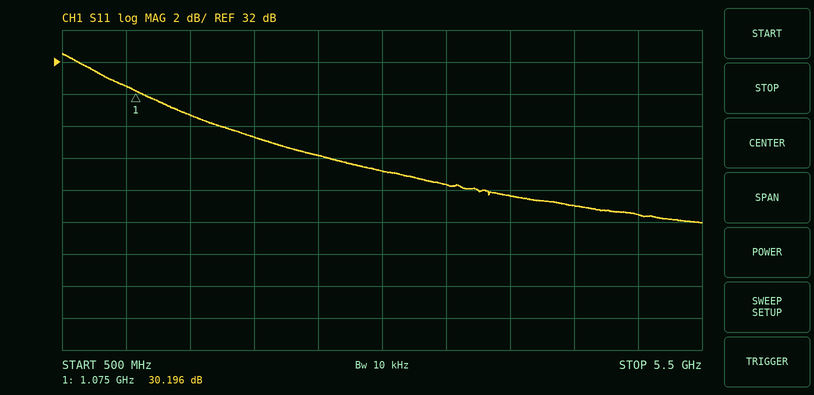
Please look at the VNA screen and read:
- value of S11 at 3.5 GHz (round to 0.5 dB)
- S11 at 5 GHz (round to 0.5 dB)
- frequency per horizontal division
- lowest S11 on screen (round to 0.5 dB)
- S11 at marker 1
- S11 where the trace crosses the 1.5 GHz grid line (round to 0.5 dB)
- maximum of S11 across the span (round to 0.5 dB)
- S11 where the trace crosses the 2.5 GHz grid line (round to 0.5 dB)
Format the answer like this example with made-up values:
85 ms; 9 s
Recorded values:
24.5 dB; 22.5 dB; 500 MHz; 22.0 dB; 30.196 dB; 28.5 dB; 32.5 dB; 26.0 dB
